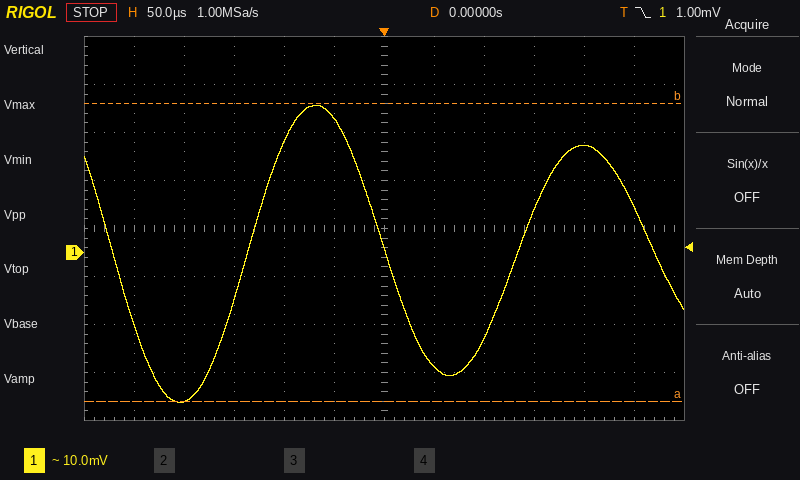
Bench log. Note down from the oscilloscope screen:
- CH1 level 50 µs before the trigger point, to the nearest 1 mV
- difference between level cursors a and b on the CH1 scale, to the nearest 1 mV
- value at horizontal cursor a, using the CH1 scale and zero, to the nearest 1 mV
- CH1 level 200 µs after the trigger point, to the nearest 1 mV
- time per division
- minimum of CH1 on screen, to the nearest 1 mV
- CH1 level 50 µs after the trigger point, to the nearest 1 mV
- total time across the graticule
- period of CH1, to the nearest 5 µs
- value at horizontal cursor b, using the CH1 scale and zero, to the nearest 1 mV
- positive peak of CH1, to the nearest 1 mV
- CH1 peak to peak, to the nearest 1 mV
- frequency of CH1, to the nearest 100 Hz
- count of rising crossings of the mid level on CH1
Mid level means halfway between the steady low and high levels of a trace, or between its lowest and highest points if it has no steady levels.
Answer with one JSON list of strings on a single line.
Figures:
["28 mV", "62 mV", "-31 mV", "22 mV", "50 µs", "-31 mV", "-24 mV", "600 µs", "270 µs", "31 mV", "31 mV", "62 mV", "3.7 kHz", "2"]
